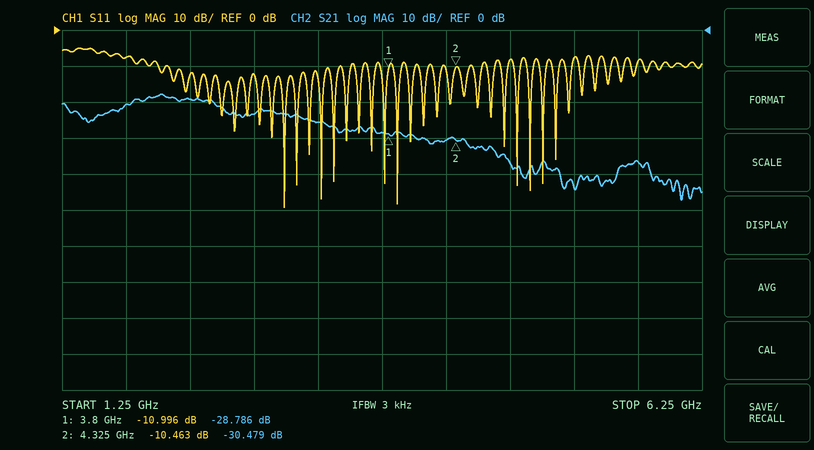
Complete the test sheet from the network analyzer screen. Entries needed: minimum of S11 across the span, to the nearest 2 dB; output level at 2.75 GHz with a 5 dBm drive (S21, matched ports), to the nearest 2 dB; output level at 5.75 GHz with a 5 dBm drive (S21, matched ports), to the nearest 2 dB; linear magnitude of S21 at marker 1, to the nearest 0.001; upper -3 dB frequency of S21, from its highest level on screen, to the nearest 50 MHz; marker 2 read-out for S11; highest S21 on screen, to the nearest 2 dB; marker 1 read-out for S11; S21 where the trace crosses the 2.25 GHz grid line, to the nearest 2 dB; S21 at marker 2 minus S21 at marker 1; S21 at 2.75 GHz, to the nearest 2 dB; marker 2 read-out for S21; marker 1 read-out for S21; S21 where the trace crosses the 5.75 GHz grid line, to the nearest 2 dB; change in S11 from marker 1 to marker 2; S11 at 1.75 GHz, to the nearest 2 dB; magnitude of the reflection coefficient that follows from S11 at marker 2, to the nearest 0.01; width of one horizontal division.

-50 dB
-18 dBm
-32 dBm
0.036
2.45 GHz
-10.463 dB
-18 dB
-10.996 dB
-20 dB
-1.693 dB
-24 dB
-30.479 dB
-28.786 dB
-36 dB
0.533 dB
-8 dB
0.30
500 MHz
